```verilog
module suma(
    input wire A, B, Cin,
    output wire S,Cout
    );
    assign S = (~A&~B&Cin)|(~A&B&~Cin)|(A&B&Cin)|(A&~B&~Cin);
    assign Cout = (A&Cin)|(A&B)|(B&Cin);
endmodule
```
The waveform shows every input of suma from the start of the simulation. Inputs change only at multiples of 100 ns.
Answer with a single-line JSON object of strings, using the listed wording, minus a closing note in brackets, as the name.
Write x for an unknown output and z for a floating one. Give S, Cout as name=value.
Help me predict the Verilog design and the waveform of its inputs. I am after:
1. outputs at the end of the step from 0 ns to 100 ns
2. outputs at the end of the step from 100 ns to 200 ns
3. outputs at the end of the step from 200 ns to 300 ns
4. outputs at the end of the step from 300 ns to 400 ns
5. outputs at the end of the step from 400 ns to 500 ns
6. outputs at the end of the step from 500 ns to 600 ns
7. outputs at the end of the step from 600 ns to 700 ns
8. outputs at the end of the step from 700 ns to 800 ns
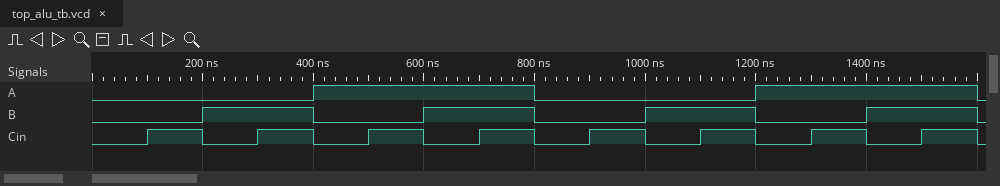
{"outputs at the end of the step from 0 ns to 100 ns": "S=0, Cout=0", "outputs at the end of the step from 100 ns to 200 ns": "S=1, Cout=0", "outputs at the end of the step from 200 ns to 300 ns": "S=1, Cout=0", "outputs at the end of the step from 300 ns to 400 ns": "S=0, Cout=1", "outputs at the end of the step from 400 ns to 500 ns": "S=1, Cout=0", "outputs at the end of the step from 500 ns to 600 ns": "S=0, Cout=1", "outputs at the end of the step from 600 ns to 700 ns": "S=0, Cout=1", "outputs at the end of the step from 700 ns to 800 ns": "S=1, Cout=1"}
